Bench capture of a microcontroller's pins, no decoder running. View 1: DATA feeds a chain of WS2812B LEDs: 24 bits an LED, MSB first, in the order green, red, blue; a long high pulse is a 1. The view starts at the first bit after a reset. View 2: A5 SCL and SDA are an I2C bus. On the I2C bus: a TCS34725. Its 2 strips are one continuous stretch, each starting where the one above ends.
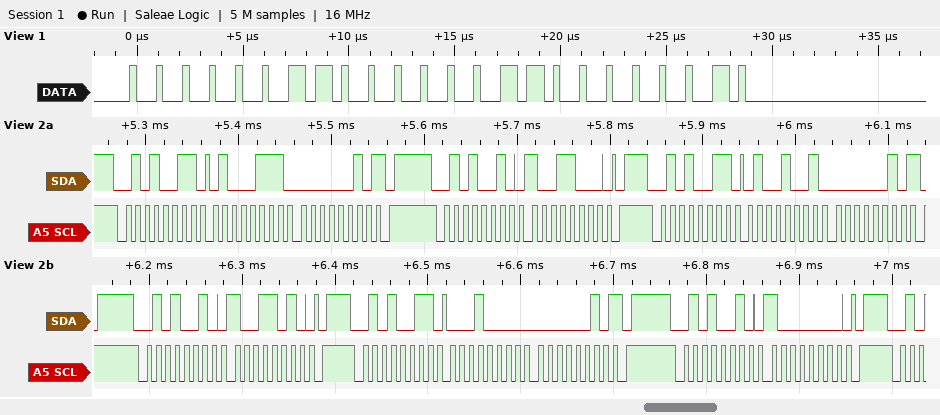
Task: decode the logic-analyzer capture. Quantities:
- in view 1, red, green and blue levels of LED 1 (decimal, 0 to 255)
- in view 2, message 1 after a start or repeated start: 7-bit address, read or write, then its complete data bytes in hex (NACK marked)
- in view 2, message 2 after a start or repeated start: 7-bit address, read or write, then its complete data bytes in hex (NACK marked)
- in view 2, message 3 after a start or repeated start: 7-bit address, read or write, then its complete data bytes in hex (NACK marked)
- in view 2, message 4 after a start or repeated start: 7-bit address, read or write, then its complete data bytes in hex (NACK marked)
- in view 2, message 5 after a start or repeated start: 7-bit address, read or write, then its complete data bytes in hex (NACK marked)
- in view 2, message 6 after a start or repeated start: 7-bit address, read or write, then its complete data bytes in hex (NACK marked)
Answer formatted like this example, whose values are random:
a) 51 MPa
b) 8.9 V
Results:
a) 3, 3, 2
b) 0x29 read: 47 02 NACK
c) 0x29 write: 98
d) 0x29 read: 49 02 NACK
e) 0x29 write: 9A
f) 0x29 read: 10 02 NACK
g) 0x29 write: 80
